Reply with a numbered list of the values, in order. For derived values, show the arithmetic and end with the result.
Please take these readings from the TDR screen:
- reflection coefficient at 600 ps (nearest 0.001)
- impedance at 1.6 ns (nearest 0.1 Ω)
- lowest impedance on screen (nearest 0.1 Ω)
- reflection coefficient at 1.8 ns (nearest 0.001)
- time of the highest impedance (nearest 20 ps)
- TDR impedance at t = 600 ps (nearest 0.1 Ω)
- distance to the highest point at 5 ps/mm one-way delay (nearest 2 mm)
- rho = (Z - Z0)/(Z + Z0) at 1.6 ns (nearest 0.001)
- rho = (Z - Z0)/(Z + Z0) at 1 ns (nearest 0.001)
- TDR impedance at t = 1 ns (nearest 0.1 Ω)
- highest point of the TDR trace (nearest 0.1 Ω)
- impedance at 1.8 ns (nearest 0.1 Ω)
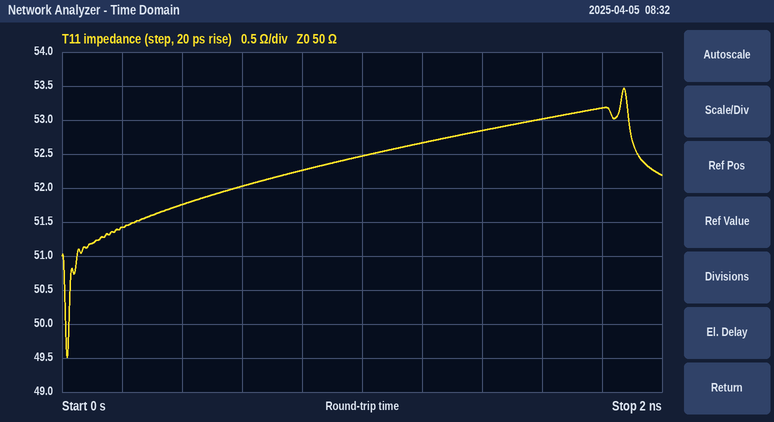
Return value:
1. (52 − 50)/(52 + 50) ≈ +0.020
2. 53.0 Ω
3. 49.5 Ω
4. (53.2 − 50)/(53.2 + 50) ≈ +0.031
5. 1.88 ns
6. 52.0 Ω
7. 1.88 ns / 2 / 5 ps/mm ≈ 188 mm
8. (53 − 50)/(53 + 50) ≈ +0.029
9. (52.5 − 50)/(52.5 + 50) ≈ +0.024
10. 52.5 Ω
11. 53.5 Ω
12. 53.2 Ω
